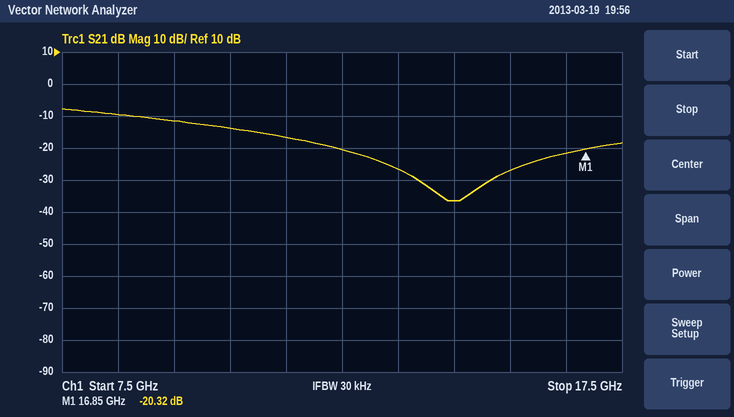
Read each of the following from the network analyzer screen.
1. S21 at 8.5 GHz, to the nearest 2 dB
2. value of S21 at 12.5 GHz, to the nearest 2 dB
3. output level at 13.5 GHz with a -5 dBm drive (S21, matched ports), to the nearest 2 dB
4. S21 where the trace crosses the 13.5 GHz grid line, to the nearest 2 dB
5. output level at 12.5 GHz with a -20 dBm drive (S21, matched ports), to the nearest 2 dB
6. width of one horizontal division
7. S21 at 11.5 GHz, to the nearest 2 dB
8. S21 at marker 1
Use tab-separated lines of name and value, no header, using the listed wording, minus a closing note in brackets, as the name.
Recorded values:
S21 at 8.5 GHz, to the nearest 2 dB	-10 dB
value of S21 at 12.5 GHz, to the nearest 2 dB	-20 dB
output level at 13.5 GHz with a -5 dBm drive (S21, matched ports), to the nearest 2 dB	-32 dBm
S21 where the trace crosses the 13.5 GHz grid line, to the nearest 2 dB	-26 dB
output level at 12.5 GHz with a -20 dBm drive (S21, matched ports), to the nearest 2 dB	-40 dBm
width of one horizontal division	1 GHz
S21 at 11.5 GHz, to the nearest 2 dB	-16 dB
S21 at marker 1	-20.32 dB
